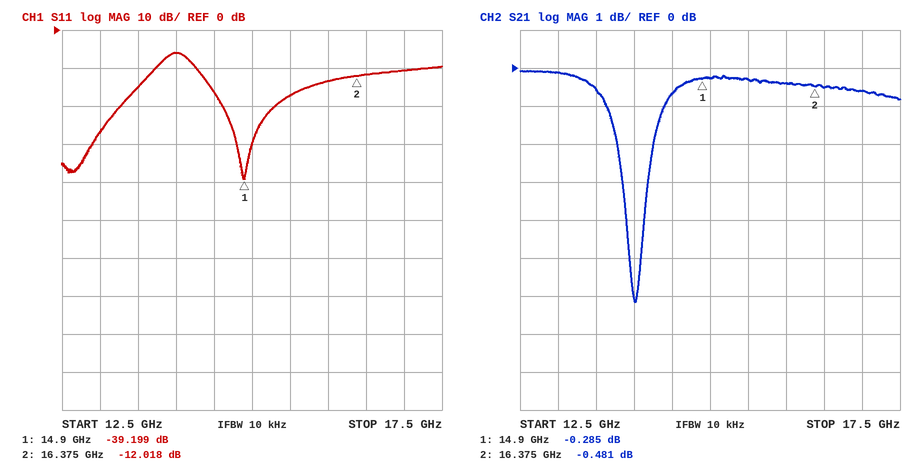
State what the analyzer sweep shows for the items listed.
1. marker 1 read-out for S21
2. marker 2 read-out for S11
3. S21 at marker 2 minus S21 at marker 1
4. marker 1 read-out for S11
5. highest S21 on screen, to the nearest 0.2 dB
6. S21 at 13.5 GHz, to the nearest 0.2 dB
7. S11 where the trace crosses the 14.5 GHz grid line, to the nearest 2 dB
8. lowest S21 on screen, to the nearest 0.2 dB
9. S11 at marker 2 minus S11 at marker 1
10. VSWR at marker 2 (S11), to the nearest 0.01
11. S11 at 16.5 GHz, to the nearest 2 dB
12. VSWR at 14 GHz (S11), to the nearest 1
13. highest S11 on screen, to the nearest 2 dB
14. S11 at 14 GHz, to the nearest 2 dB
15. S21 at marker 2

-0.285 dB
-12.018 dB
-0.196 dB
-39.199 dB
0.0 dB
-0.6 dB
-16 dB
-6.2 dB
27.181 dB
1.67
-12 dB
3
-6 dB
-6 dB
-0.481 dB
